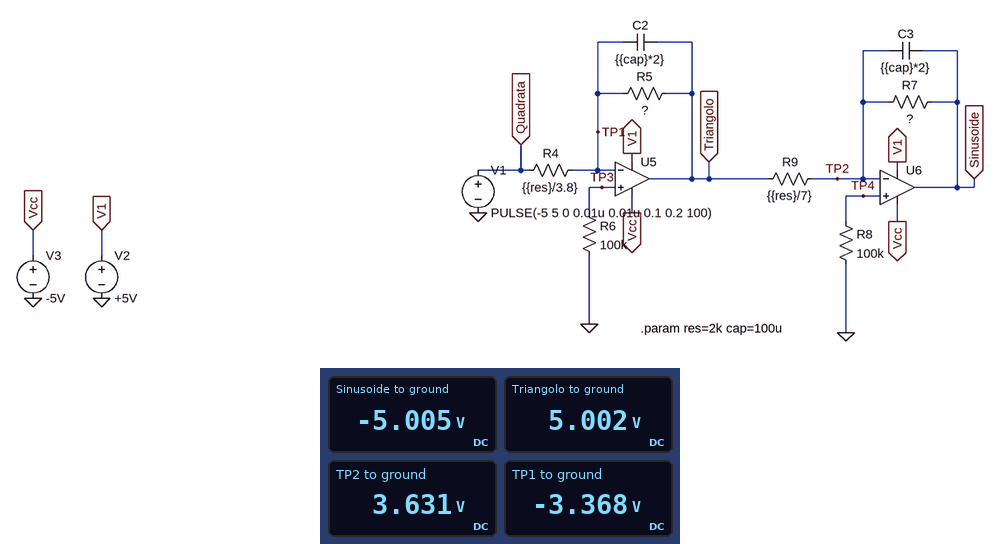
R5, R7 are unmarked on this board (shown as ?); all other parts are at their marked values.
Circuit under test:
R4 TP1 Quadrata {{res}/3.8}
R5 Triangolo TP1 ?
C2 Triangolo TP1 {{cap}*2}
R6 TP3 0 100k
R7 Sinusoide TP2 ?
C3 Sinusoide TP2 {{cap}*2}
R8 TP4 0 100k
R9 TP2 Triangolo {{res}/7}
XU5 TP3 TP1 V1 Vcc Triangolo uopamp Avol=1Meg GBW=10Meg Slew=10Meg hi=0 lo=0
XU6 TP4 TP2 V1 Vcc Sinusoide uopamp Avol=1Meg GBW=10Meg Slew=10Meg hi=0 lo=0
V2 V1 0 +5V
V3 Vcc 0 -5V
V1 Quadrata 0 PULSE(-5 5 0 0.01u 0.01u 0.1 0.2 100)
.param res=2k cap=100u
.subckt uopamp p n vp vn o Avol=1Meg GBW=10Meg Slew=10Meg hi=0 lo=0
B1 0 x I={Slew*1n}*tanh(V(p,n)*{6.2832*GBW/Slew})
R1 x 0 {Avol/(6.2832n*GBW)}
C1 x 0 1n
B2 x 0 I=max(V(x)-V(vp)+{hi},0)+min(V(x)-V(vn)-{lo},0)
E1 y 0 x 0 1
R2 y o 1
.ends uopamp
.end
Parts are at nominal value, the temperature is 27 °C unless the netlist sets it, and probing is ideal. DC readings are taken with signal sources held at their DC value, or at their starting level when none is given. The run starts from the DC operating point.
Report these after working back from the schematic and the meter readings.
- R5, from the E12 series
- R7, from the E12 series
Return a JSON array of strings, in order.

["2.7 kΩ", "1.8 kΩ"]
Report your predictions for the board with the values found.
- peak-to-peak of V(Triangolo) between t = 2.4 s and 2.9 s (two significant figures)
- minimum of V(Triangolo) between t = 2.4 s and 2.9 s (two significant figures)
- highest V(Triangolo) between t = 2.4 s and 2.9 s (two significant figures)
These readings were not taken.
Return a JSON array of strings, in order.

["4.8 V", "-2.4 V", "2.4 V"]
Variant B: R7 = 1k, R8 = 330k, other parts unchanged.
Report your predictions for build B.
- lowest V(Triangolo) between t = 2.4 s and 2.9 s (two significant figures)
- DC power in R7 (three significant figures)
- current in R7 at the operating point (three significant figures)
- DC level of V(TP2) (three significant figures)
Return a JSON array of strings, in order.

["-2.4 V", "60.5 mW", "7.78 mA", "2.78 V"]
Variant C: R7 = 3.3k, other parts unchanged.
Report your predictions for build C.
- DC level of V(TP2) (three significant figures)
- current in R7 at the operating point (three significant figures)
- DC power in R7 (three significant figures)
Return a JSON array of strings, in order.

["4.21 V", "2.79 mA", "25.7 mW"]
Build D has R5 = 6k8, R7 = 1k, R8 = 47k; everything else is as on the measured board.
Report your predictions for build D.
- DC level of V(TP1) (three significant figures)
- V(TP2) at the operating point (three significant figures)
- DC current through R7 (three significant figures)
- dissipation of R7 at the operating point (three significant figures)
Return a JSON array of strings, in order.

["-4.28 V", "2.78 V", "7.78 mA", "60.5 mW"]
